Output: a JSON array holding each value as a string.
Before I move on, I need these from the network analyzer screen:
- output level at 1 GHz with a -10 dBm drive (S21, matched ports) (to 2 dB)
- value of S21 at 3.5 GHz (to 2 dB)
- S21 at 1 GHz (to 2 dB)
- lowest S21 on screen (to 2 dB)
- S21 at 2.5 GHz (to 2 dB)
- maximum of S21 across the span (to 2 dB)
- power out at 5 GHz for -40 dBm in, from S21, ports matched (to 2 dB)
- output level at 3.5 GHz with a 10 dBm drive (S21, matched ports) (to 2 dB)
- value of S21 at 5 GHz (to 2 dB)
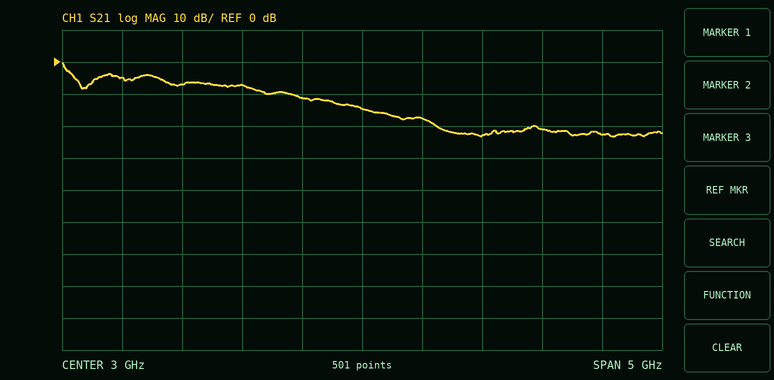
["-14 dBm", "-18 dB", "-4 dB", "-24 dB", "-12 dB", "0 dB", "-62 dBm", "-8 dBm", "-22 dB"]
